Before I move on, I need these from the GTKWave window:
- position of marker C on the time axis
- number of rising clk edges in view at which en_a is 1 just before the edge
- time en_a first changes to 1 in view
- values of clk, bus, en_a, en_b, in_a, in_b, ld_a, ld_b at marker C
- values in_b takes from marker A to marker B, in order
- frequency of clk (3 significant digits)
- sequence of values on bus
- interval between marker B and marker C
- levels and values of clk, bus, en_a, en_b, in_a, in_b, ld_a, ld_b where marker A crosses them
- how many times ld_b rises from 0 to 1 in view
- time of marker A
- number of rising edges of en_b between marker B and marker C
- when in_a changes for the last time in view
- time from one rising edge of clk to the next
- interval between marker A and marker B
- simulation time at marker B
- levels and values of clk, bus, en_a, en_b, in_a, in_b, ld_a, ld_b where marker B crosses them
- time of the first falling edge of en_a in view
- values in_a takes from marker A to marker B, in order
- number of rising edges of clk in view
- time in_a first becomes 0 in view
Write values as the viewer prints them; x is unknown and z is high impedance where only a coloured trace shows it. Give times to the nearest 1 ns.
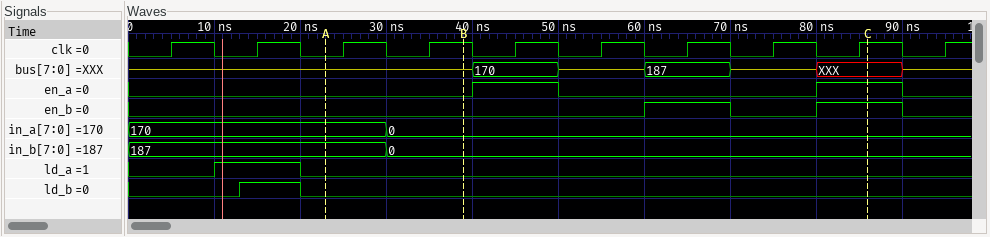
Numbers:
86 ns
2
40 ns
clk=1, bus=XXX, en_a=1, en_b=1, in_a=0, in_b=0, ld_a=0, ld_b=0
187, 0
100 MHz
z, 170, z, 187, z, XXX, z
47 ns
clk=0, bus=z, en_a=0, en_b=0, in_a=170, in_b=187, ld_a=0, ld_b=0
1
23 ns
2
30 ns
10 ns
16 ns
39 ns
clk=1, bus=z, en_a=0, en_b=0, in_a=0, in_b=0, ld_a=0, ld_b=0
50 ns
170, 0
10
30 ns
